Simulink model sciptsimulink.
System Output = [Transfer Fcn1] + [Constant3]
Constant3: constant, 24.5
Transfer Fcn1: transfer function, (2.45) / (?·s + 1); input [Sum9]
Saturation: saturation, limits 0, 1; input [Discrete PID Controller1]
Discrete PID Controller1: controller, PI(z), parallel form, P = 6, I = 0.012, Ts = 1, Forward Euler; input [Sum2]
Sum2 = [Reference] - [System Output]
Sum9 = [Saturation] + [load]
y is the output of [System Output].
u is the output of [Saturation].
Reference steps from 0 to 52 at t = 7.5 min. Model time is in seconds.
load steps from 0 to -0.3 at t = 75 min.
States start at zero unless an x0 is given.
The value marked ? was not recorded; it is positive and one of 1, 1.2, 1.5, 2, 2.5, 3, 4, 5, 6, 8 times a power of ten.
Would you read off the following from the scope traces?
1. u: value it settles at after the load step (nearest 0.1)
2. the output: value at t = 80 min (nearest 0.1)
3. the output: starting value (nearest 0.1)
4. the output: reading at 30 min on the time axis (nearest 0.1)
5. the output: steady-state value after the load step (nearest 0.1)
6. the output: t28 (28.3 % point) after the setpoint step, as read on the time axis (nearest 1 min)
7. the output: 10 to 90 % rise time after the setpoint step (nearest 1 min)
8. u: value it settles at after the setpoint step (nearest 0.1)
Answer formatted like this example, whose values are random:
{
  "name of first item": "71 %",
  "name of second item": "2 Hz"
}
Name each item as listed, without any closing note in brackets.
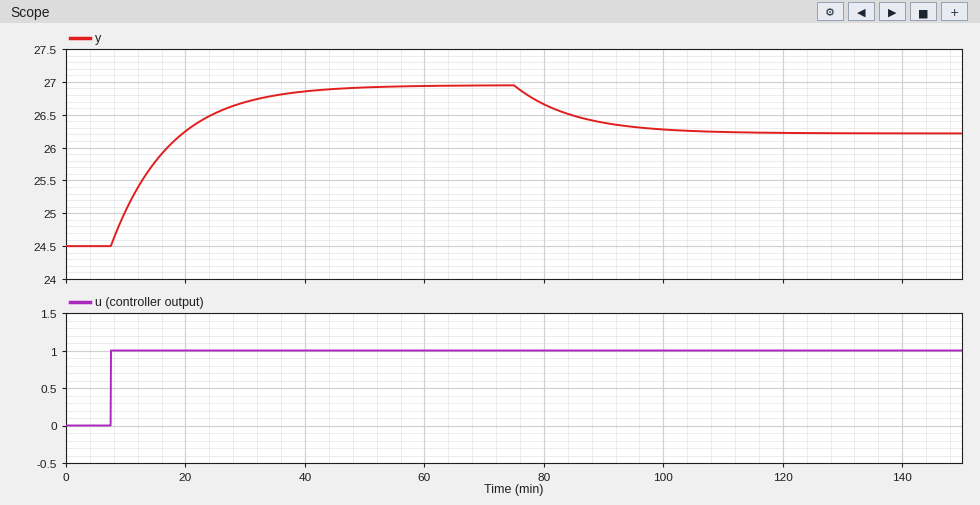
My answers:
{
  "u: value it settles at after the load step": "1.0",
  "the output: value at t = 80 min": "26.7",
  "the output: starting value": "24.5",
  "the output: reading at 30 min on the time axis": "26.7",
  "the output: steady-state value after the load step": "26.2",
  "the output: t28 (28.3 % point) after the setpoint step, as read on the time axis": "11 min",
  "the output: 10 to 90 % rise time after the setpoint step": "22 min",
  "u: value it settles at after the setpoint step": "1.0"
}
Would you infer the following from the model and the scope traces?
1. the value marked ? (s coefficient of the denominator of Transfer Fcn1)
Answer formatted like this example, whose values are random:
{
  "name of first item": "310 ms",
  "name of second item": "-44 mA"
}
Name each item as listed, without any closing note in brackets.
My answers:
{
  "the value marked ?": "600"
}
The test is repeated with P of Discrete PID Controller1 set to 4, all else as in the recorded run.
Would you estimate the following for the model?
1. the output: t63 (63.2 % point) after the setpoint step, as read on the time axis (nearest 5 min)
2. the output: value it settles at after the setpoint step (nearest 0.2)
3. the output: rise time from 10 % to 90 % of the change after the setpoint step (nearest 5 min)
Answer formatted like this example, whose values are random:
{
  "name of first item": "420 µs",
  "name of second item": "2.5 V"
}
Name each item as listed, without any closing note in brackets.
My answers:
{
  "the output: t63 (63.2 % point) after the setpoint step, as read on the time axis": "20 min",
  "the output: value it settles at after the setpoint step": "27.0",
  "the output: rise time from 10 % to 90 % of the change after the setpoint step": "20 min"
}
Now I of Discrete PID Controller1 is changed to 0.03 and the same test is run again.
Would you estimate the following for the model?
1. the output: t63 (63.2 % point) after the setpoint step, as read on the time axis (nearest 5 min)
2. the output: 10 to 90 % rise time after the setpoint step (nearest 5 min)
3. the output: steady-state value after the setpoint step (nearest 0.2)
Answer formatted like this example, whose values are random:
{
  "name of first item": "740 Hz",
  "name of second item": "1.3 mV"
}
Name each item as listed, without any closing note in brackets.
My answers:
{
  "the output: t63 (63.2 % point) after the setpoint step, as read on the time axis": "20 min",
  "the output: 10 to 90 % rise time after the setpoint step": "20 min",
  "the output: steady-state value after the setpoint step": "27.0"
}
